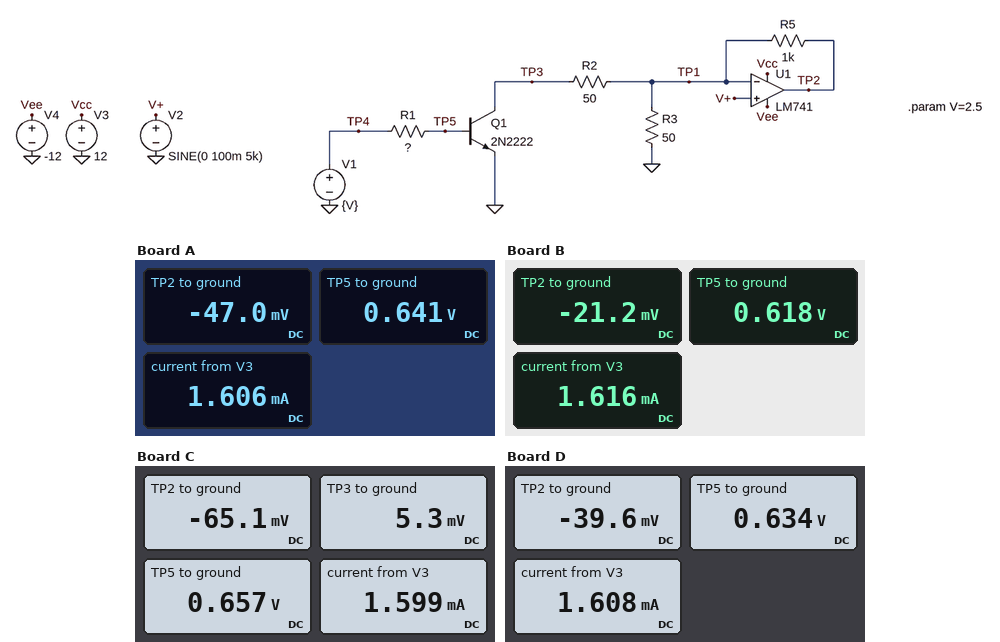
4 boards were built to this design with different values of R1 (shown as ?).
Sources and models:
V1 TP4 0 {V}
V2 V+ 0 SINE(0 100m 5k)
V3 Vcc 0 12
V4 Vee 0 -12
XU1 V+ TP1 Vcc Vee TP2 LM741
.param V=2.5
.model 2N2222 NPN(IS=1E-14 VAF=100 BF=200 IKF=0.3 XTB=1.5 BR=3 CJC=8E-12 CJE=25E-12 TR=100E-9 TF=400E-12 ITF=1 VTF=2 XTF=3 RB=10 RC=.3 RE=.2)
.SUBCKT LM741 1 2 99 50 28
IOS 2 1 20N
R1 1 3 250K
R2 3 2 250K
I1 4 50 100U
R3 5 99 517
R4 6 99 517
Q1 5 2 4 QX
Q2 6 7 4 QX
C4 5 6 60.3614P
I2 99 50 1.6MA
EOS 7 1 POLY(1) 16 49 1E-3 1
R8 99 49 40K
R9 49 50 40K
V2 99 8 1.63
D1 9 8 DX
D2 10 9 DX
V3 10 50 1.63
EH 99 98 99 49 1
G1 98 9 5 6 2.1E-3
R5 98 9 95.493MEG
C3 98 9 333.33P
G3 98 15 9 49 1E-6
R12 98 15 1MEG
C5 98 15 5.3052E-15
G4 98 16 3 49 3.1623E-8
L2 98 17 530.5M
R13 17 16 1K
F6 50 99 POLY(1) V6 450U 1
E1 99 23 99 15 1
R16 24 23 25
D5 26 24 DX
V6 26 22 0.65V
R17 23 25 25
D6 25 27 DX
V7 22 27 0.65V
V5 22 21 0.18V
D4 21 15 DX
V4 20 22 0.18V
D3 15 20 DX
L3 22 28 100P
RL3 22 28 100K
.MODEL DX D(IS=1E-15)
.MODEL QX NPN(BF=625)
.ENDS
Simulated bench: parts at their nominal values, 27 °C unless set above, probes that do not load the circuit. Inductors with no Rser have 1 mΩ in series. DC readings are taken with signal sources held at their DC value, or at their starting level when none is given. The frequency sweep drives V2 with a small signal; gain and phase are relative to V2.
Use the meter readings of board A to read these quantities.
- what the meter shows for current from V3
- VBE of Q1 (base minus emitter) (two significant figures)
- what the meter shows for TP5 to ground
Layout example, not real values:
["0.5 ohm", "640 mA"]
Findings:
["1.606 mA", "640 mV", "0.641 V"]
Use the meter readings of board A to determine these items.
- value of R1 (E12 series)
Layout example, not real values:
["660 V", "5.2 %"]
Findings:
["12 kΩ"]
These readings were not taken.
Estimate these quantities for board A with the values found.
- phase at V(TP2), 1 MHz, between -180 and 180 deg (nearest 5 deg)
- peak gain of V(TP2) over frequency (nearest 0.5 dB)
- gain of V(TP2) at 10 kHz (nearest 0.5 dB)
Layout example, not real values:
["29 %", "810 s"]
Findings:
["-110 deg", "30.0 dB", "29.5 dB"]
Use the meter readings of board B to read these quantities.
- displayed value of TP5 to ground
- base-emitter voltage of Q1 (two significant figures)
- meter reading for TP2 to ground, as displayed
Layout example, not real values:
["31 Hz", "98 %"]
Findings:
["0.618 V", "620 mV", "-21.2 mV"]
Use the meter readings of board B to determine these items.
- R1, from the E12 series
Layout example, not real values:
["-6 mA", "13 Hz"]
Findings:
["27 kΩ"]
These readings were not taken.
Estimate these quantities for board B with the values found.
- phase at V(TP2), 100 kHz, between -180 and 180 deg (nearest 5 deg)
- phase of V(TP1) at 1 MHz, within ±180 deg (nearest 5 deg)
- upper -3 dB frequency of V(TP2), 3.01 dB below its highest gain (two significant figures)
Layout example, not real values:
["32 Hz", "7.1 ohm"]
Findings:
["-75 deg", "-110 deg", "32 kHz"]
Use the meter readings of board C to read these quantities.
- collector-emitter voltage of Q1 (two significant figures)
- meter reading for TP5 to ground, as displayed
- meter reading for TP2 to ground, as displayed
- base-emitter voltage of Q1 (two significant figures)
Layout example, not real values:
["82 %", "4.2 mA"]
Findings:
["5.3 mV", "0.657 V", "-65.1 mV", "660 mV"]
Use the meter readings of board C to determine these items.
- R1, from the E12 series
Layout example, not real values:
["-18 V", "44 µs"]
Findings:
["6.8 kΩ"]
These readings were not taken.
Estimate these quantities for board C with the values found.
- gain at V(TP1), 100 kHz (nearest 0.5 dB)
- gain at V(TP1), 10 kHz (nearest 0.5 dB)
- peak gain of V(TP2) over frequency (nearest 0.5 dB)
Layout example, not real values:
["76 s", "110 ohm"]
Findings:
["-12.0 dB", "-0.5 dB", "30.5 dB"]
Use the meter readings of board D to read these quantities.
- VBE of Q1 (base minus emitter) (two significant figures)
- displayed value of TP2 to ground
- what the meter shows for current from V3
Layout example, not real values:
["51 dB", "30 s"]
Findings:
["630 mV", "-39.6 mV", "1.608 mA"]
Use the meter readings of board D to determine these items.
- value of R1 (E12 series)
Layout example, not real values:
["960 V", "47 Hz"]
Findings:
["15 kΩ"]
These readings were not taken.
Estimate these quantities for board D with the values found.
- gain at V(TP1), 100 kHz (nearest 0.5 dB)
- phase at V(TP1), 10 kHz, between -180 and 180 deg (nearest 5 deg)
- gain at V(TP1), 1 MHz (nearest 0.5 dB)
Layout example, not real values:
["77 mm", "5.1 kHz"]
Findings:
["-11.0 dB", "-20 deg", "-31.5 dB"]
